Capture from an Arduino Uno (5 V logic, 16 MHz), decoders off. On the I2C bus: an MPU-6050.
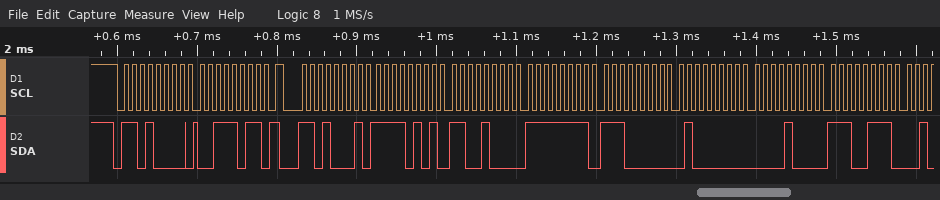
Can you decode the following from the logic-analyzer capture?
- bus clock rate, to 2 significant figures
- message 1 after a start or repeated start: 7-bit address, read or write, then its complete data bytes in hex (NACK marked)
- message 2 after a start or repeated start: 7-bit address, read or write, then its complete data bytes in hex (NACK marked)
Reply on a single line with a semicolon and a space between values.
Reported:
100 kHz; 0x68 write: 3B; 0x68 read: F5 C8 FF E0 40 08 E7
